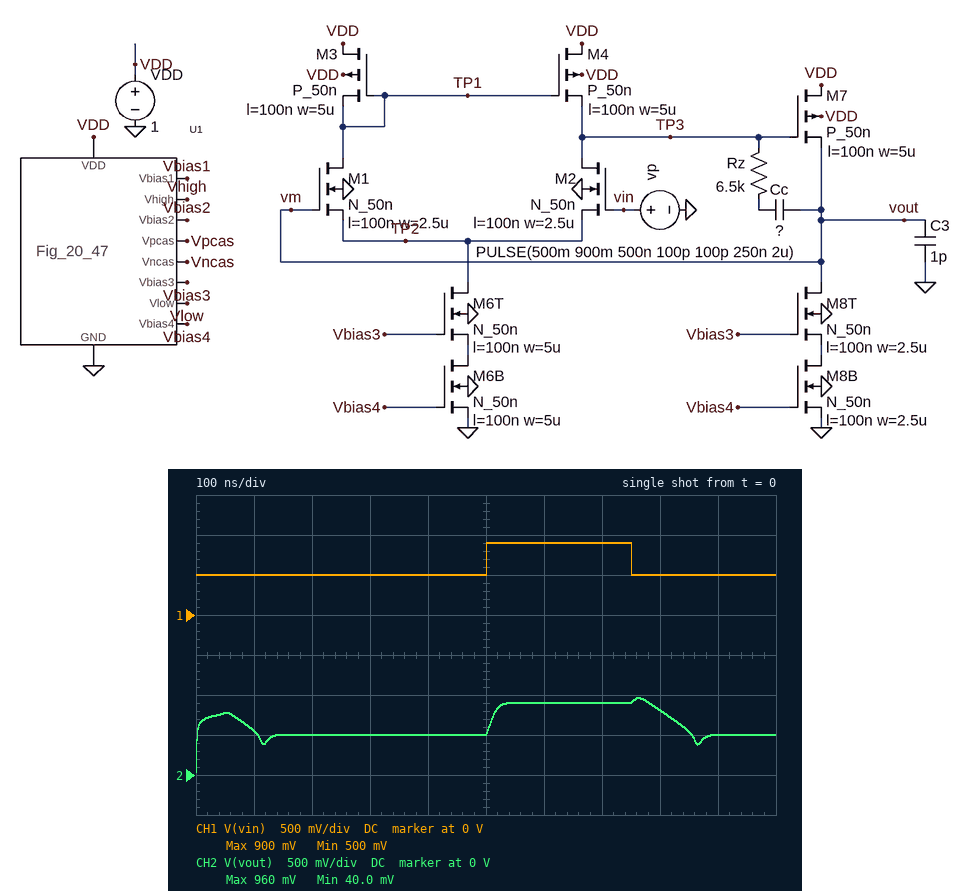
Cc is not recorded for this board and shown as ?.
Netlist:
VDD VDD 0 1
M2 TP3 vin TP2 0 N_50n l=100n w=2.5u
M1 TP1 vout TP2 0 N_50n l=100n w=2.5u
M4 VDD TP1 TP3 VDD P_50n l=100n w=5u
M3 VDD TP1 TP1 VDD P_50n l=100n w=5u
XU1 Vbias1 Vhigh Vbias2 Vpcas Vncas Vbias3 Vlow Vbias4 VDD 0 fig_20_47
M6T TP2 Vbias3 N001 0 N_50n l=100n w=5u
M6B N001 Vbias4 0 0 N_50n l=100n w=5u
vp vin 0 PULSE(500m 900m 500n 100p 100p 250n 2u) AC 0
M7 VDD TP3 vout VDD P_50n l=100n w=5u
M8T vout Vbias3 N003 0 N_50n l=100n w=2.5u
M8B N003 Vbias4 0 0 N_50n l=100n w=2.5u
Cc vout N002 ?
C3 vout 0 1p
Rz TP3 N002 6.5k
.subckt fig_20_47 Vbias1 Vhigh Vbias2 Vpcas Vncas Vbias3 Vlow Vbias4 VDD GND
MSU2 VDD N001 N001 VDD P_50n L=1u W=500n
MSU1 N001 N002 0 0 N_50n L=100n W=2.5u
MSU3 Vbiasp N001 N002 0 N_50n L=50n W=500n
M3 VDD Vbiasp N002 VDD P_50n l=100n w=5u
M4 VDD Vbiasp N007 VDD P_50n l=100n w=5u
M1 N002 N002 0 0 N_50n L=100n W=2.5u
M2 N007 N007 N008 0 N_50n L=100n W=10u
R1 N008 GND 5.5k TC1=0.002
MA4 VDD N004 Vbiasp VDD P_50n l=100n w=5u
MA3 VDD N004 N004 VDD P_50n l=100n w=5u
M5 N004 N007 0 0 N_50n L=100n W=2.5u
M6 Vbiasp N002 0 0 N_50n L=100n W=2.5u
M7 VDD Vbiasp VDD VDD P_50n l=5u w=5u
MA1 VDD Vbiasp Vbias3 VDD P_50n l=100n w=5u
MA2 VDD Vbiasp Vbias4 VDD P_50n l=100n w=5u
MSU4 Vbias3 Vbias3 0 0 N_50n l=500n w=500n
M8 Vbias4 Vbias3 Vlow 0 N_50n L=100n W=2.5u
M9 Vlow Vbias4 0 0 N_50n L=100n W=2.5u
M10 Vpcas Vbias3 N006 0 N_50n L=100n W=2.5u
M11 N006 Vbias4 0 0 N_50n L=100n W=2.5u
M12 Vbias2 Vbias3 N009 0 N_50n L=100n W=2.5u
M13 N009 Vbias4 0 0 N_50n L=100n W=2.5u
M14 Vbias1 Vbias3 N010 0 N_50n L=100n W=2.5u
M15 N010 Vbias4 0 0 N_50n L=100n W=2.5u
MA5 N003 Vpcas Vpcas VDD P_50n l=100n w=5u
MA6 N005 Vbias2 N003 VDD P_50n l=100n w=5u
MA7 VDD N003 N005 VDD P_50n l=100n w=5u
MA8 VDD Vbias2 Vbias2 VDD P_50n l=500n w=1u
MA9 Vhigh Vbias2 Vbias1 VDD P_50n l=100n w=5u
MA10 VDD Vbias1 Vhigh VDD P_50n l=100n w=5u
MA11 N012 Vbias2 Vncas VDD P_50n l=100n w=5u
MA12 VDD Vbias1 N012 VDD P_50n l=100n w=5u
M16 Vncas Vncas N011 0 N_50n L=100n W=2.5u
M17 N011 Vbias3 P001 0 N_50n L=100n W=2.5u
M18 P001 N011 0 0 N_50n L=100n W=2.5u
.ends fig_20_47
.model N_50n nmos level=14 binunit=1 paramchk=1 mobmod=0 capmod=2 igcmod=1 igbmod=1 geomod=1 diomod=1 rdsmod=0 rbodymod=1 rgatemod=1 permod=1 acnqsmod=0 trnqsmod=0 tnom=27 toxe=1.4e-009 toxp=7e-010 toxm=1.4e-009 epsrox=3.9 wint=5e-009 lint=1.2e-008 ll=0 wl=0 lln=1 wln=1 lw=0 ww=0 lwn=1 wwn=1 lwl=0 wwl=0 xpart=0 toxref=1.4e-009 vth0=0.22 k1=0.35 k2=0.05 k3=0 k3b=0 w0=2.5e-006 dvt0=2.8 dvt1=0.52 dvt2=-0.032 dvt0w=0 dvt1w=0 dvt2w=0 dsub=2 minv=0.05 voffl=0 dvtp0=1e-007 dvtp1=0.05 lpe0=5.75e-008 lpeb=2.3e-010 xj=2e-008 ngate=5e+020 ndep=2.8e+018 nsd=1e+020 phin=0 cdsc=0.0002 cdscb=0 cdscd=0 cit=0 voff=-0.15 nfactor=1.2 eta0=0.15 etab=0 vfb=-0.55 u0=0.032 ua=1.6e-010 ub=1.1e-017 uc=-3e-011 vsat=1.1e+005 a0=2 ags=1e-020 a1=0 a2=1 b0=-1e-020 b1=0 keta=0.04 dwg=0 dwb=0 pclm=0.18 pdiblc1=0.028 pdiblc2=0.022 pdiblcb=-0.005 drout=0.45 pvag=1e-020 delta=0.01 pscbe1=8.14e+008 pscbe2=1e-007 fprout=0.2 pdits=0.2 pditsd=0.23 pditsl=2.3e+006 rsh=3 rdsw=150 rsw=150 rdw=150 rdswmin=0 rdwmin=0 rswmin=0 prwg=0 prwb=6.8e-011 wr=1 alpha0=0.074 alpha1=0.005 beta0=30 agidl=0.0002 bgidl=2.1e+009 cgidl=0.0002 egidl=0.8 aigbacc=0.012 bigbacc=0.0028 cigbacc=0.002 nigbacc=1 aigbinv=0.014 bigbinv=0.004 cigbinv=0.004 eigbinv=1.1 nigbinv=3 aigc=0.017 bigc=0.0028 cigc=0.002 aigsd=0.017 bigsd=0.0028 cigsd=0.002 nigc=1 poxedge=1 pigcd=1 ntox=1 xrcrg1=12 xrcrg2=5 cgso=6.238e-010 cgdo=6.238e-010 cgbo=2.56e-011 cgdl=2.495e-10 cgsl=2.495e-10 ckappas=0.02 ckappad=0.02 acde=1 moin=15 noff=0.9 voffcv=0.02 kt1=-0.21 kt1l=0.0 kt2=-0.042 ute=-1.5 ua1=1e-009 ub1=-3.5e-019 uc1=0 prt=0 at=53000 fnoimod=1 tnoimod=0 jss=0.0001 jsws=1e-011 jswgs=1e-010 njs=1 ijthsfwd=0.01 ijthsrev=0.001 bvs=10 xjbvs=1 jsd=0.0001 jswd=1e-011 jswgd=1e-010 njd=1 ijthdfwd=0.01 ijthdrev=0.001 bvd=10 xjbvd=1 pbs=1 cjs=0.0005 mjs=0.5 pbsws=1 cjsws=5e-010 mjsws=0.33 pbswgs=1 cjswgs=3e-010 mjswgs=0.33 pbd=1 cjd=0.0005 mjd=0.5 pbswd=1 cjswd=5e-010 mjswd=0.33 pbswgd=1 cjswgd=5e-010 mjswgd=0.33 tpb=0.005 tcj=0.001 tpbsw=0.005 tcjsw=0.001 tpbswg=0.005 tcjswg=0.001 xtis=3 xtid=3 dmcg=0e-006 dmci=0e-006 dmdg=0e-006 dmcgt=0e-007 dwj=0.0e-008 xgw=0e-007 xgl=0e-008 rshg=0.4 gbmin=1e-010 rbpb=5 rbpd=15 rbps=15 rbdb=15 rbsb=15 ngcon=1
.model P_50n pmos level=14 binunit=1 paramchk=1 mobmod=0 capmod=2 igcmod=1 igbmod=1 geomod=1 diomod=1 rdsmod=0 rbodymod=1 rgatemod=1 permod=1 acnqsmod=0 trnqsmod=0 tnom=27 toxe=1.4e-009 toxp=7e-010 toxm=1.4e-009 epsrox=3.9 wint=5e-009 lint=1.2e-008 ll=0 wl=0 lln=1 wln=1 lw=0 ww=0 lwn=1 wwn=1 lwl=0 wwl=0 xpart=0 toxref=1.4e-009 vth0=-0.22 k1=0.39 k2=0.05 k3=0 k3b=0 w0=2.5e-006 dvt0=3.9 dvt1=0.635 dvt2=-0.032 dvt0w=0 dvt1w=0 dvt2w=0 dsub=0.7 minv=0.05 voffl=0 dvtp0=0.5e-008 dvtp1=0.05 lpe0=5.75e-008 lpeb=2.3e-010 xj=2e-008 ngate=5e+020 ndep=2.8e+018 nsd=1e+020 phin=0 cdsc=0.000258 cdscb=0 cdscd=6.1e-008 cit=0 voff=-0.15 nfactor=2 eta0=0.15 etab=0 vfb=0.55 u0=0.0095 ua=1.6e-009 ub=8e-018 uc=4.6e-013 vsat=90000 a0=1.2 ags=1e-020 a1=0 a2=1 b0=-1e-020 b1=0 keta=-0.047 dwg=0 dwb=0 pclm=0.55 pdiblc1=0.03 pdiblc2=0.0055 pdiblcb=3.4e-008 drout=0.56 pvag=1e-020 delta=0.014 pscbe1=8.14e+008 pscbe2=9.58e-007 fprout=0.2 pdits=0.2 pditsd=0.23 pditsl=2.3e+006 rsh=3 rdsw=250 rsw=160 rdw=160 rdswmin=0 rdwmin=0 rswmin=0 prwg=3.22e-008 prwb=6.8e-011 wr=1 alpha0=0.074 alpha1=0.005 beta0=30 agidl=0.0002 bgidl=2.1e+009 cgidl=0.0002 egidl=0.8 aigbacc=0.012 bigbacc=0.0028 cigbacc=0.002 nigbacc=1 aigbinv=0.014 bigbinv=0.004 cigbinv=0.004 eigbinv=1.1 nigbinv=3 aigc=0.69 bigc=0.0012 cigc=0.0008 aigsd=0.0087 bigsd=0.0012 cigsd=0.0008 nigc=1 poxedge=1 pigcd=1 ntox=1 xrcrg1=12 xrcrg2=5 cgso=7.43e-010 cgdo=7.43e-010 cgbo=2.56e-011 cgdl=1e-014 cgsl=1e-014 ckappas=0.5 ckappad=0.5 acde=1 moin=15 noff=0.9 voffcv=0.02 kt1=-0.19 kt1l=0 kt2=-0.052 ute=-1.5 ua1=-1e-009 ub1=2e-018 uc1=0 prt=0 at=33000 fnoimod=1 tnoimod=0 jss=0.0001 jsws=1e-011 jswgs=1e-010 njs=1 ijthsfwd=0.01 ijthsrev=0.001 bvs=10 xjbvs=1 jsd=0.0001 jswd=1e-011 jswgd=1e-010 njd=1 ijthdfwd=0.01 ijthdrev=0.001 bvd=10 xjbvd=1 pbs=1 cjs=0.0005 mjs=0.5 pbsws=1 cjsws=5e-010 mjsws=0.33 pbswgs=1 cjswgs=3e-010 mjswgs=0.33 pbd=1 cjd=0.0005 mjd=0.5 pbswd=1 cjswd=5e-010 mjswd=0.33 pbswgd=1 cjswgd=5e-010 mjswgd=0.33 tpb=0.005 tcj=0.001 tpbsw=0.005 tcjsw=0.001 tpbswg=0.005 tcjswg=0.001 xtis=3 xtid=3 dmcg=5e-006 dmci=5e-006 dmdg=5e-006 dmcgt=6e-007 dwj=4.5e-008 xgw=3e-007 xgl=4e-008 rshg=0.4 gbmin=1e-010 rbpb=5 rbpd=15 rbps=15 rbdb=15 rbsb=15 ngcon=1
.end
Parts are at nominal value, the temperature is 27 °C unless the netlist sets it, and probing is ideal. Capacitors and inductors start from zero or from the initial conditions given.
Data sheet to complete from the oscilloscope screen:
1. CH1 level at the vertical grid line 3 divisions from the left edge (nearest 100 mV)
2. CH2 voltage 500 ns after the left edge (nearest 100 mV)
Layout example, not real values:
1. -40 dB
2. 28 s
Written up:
1. 500 mV
2. 500 mV
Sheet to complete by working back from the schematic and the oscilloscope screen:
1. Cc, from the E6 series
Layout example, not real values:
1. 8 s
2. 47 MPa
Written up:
1. 1 pF
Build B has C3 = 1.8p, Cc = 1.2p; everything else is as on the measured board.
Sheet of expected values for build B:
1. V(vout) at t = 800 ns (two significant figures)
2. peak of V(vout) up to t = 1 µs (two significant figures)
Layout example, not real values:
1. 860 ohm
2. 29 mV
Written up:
1. 860 mV
2. 950 mV
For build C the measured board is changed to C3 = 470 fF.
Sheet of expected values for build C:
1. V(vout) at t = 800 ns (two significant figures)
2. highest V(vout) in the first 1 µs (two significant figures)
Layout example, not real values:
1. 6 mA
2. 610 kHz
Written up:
1. 760 mV
2. 1.0 V
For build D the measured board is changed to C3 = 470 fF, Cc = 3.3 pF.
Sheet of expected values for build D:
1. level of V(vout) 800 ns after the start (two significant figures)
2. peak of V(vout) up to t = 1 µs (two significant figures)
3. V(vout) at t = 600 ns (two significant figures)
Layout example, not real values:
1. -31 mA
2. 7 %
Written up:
1. 1.0 V
2. 1.1 V
3. 880 mV
